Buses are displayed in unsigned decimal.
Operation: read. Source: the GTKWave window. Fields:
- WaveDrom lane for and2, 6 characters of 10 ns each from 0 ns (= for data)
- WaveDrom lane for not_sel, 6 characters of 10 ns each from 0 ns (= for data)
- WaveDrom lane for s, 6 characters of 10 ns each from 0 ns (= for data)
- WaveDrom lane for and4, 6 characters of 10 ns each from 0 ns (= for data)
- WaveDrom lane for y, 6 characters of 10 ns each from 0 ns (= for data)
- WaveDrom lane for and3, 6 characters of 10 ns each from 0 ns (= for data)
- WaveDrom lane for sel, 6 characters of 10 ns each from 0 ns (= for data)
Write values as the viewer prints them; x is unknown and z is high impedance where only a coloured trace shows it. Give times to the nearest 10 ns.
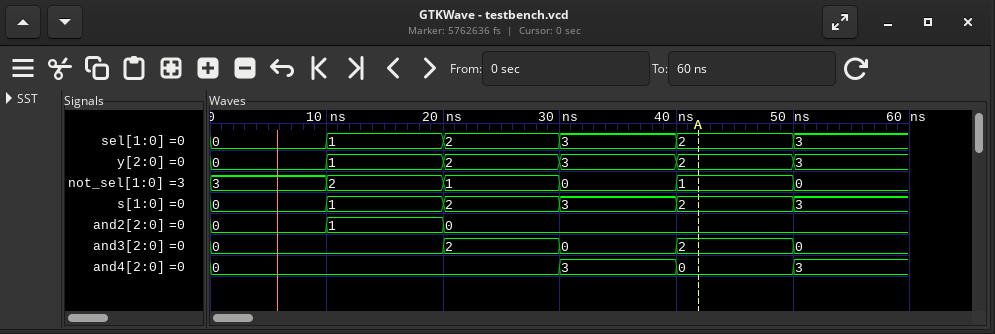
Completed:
{name: 'and2', wave: '===...', data: '0 1 0'}
{name: 'not_sel', wave: '======', data: '3 2 1 0 1 0'}
{name: 's', wave: '======', data: '0 1 2 3 2 3'}
{name: 'and4', wave: '=..===', data: '0 3 0 3'}
{name: 'y', wave: '======', data: '0 1 2 3 2 3'}
{name: 'and3', wave: '=.====', data: '0 2 0 2 0'}
{name: 'sel', wave: '======', data: '0 1 2 3 2 3'}
